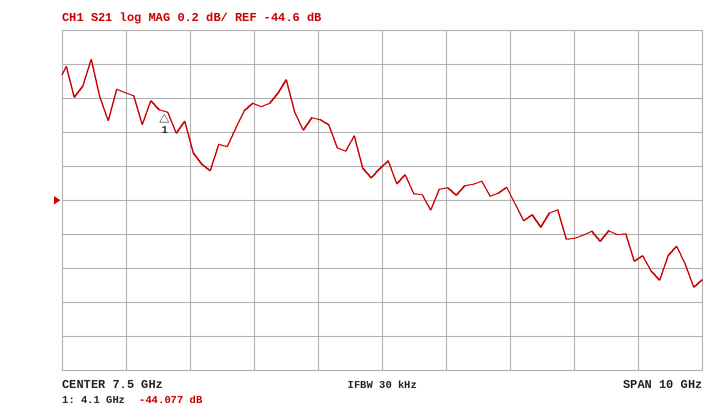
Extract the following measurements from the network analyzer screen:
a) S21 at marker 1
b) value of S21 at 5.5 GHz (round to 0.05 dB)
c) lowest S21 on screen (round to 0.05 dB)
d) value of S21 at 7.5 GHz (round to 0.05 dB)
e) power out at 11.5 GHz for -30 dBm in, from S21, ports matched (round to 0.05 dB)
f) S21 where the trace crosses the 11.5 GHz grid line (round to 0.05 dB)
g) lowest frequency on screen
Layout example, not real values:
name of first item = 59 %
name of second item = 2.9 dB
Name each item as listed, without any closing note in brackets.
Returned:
S21 at marker 1 = -44.077 dB
value of S21 at 5.5 GHz = -44.05 dB
lowest S21 on screen = -45.10 dB
value of S21 at 7.5 GHz = -44.40 dB
power out at 11.5 GHz for -30 dBm in, from S21, ports matched = -74.95 dBm
S21 where the trace crosses the 11.5 GHz grid line = -44.95 dB
lowest frequency on screen = 2.5 GHz
